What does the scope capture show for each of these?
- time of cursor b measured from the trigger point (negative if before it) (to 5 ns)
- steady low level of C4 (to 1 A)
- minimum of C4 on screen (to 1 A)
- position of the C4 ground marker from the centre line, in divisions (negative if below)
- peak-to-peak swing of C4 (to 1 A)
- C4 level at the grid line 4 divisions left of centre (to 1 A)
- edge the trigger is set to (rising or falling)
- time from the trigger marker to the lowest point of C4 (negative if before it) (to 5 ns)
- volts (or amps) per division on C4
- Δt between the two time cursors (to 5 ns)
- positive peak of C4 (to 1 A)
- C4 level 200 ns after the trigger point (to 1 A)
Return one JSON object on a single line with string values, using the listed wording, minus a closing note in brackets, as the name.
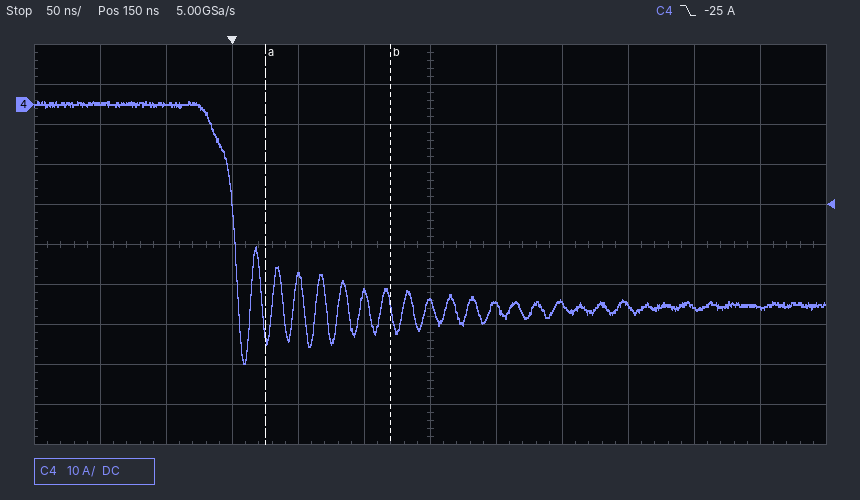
{"time of cursor b measured from the trigger point (negative if before it)": "+120 ns", "steady low level of C4": "-50 A", "minimum of C4 on screen": "-65 A", "position of the C4 ground marker from the centre line, in divisions": "+3.5 div", "peak-to-peak swing of C4": "66 A", "C4 level at the grid line 4 divisions left of centre": "0 A", "edge the trigger is set to": "falling", "time from the trigger marker to the lowest point of C4 (negative if before it)": "+10 ns", "volts (or amps) per division on C4": "10 A", "Δt between the two time cursors": "95 ns", "positive peak of C4": "1 A", "C4 level 200 ns after the trigger point": "-50 A"}
